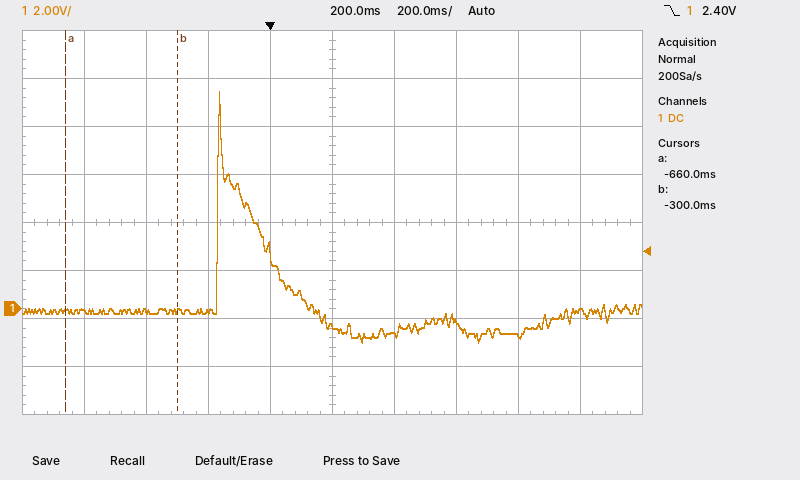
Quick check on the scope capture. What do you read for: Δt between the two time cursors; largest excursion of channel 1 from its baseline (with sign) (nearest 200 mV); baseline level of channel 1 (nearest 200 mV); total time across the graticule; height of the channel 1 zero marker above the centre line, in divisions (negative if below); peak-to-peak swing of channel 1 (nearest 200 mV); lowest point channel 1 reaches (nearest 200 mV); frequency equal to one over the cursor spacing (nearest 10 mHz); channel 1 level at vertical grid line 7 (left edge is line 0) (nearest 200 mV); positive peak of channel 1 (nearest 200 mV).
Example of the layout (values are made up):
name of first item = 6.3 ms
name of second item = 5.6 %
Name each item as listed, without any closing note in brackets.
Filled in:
Δt between the two time cursors = 360 ms
largest excursion of channel 1 from its baseline (with sign) = +9.2 V
baseline level of channel 1 = -200 mV
total time across the graticule = 2 s
height of the channel 1 zero marker above the centre line, in divisions = -1.8 div
peak-to-peak swing of channel 1 = 10.4 V
lowest point channel 1 reaches = -1.4 V
frequency equal to one over the cursor spacing = 2.78 Hz
channel 1 level at vertical grid line 7 (left edge is line 0) = -600 mV
positive peak of channel 1 = 9.0 V
